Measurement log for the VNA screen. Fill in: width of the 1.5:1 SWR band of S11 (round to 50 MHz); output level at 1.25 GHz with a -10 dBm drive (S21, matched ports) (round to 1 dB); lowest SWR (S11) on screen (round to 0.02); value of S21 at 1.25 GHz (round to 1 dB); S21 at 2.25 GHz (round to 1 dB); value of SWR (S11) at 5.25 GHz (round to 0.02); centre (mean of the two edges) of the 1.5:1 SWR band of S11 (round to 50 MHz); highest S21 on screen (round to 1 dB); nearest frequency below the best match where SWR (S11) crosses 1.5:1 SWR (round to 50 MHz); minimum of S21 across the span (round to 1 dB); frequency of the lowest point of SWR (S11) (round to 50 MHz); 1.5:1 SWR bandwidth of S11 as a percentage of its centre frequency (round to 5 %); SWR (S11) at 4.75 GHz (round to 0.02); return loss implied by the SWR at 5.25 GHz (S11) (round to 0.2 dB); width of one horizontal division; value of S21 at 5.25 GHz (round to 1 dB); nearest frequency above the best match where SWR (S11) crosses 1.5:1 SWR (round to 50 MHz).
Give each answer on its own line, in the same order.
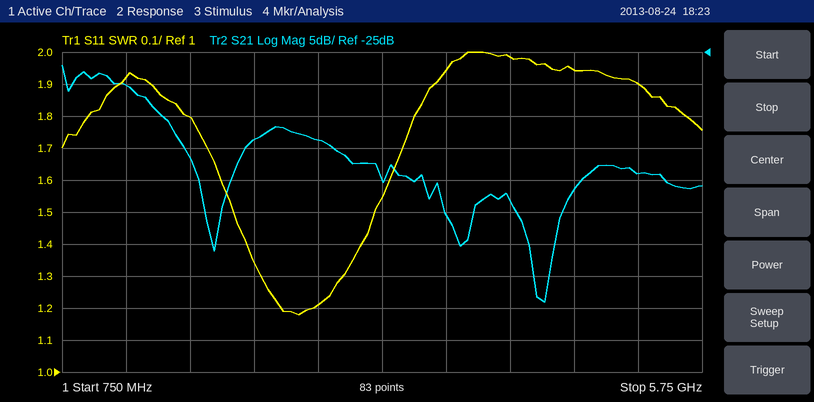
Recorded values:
1.10 GHz
-40 dBm
1.18
-30 dB
-39 dB
1.90
2.65 GHz
-27 dB
2.10 GHz
-64 dB
2.60 GHz
40 %
1.94
10.2 dB
500 MHz
-44 dB
3.20 GHz
